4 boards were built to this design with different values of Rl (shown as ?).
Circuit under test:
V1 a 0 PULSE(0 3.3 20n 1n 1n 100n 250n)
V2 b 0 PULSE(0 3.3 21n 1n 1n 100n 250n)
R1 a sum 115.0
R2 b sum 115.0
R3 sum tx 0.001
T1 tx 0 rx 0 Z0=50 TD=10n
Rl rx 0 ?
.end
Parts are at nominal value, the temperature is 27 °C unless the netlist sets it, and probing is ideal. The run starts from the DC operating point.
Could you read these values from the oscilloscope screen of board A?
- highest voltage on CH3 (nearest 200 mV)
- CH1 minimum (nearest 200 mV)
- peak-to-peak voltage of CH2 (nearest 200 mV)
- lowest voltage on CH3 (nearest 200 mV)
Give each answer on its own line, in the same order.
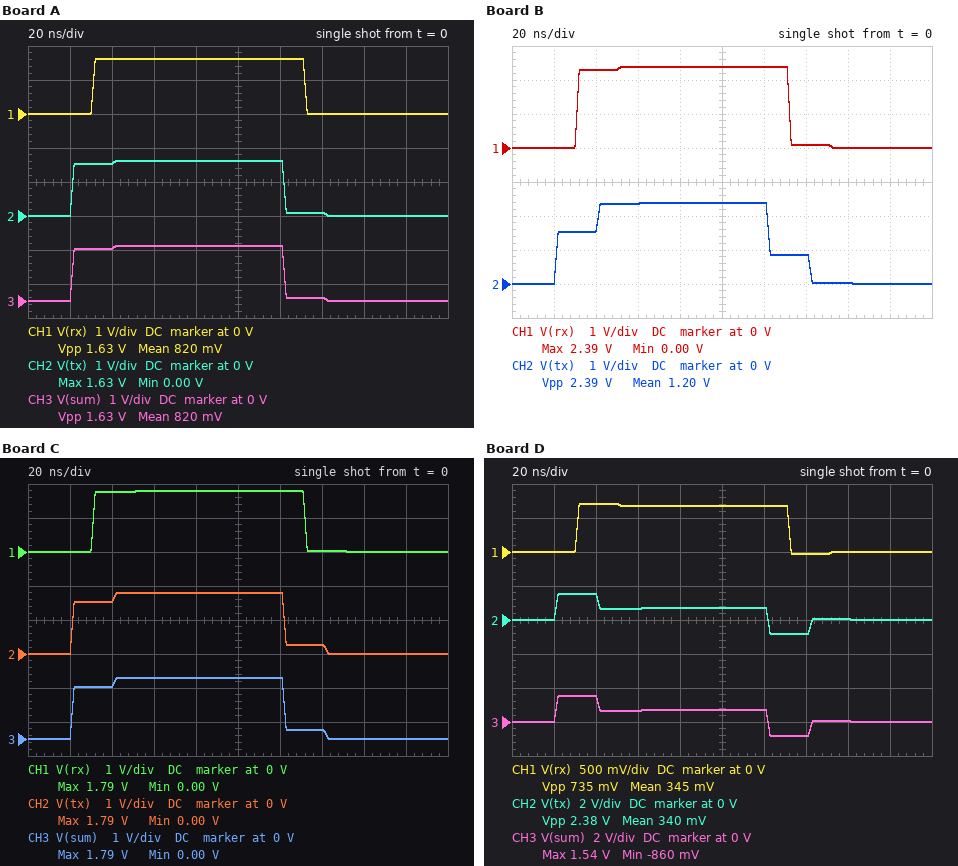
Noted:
1.6 V
0 V
1.6 V
0 V
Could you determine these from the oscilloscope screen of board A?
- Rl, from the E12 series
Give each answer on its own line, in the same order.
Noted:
56 Ω
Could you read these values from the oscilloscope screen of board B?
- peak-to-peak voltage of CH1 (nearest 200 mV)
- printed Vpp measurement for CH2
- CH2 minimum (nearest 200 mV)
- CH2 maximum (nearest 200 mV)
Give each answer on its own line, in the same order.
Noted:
2.4 V
2.39 V
0 V
2.4 V
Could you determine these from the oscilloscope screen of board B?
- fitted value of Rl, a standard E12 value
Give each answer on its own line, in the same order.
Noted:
150 Ω
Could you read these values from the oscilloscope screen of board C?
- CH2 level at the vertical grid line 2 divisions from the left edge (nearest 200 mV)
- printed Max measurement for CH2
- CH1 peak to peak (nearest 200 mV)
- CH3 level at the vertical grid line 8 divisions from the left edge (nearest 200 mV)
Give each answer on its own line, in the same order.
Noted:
1.6 V
1.79 V
1.8 V
0 V
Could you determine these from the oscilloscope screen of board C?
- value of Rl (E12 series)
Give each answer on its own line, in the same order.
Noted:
68 Ω
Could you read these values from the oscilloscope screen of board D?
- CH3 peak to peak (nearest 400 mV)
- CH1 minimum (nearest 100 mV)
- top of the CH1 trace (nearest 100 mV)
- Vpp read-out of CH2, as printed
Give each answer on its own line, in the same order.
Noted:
2.4 V
0 V
700 mV
2.38 V
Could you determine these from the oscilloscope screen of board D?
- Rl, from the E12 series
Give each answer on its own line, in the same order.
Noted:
15 Ω
